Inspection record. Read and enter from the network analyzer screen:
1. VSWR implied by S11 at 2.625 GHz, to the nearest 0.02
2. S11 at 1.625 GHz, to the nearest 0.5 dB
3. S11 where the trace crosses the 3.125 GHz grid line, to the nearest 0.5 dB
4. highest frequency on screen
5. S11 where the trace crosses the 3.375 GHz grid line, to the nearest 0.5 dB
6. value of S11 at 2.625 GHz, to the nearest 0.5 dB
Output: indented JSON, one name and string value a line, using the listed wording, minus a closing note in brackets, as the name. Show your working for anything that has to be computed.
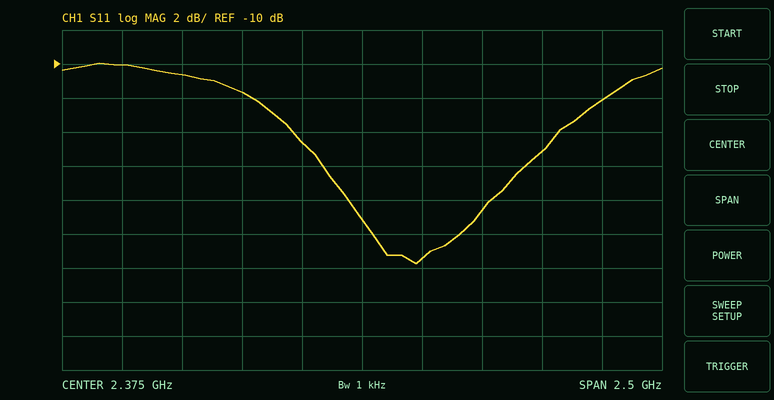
{
  "VSWR implied by S11 at 2.625 GHz, to the nearest 0.02": "|Γ| = 10^(-21.5/20) = 0.0841; VSWR = (1 + 0.0841)/(1 − 0.0841) ≈ 1.18",
  "S11 at 1.625 GHz, to the nearest 0.5 dB": "-10.5 dB",
  "S11 where the trace crosses the 3.125 GHz grid line, to the nearest 0.5 dB": "-15.0 dB",
  "highest frequency on screen": "3.625 GHz",
  "S11 where the trace crosses the 3.375 GHz grid line, to the nearest 0.5 dB": "-12.0 dB",
  "value of S11 at 2.625 GHz, to the nearest 0.5 dB": "-21.5 dB"
}
